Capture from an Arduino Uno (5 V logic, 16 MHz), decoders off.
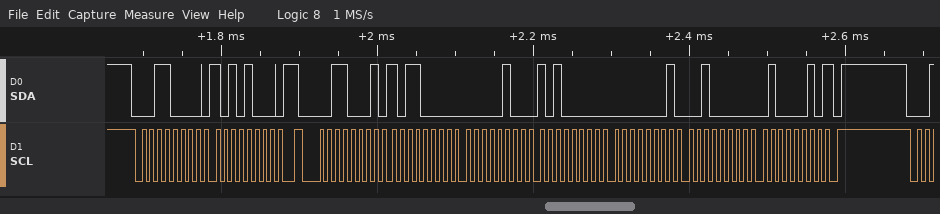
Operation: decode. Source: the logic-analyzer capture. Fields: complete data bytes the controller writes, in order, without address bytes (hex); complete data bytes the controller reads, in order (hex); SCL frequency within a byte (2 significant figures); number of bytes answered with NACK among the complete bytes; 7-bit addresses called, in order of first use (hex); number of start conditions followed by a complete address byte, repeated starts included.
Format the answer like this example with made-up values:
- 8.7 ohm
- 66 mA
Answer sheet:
- A8
- B0 04 A0 01 20 42
- 100 kHz
- 1
- 0x18
- 2
